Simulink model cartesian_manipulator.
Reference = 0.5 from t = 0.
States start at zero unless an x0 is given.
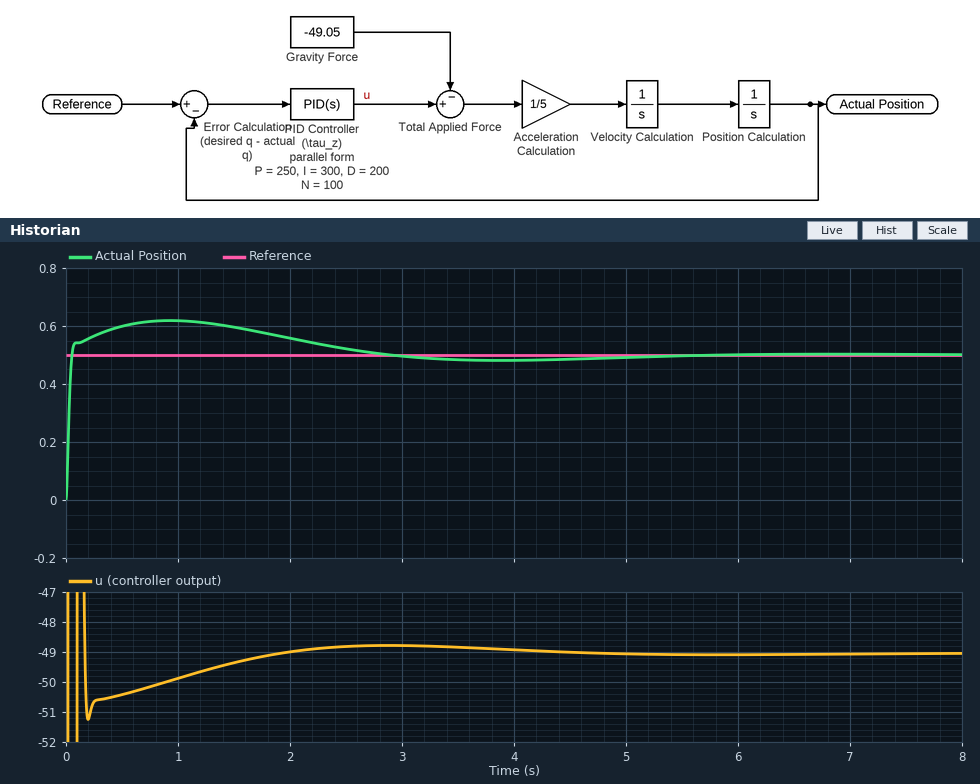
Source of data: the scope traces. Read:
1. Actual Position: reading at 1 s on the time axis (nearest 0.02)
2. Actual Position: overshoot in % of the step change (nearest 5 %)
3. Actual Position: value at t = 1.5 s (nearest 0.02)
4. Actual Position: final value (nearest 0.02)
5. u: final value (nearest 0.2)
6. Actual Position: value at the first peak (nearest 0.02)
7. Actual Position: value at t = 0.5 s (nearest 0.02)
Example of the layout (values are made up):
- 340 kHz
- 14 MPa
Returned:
- 0.62
- 25 %
- 0.60
- 0.50
- -49.0
- 0.62
- 0.60
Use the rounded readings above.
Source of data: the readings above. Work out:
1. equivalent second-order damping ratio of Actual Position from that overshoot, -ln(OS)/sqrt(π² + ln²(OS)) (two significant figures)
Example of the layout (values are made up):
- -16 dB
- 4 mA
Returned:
- 0.40
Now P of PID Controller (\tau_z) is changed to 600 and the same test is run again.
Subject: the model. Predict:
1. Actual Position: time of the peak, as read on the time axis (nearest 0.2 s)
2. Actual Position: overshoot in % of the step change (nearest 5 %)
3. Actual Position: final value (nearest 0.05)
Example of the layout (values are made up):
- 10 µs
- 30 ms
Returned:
- 0.6 s
- 15 %
- 0.50
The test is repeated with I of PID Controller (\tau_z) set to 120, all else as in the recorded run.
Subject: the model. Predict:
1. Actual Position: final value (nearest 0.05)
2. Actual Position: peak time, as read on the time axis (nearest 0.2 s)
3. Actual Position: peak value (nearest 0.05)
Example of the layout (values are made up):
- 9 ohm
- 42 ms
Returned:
- 0.50
- 1.4 s
- 0.65
